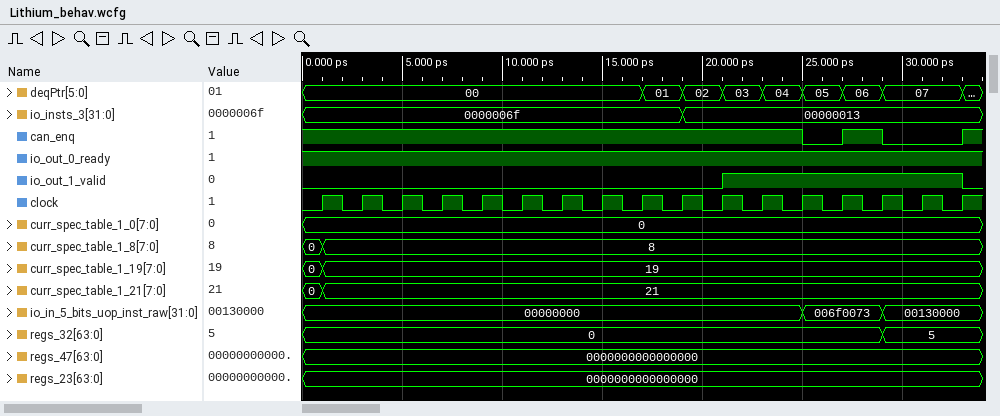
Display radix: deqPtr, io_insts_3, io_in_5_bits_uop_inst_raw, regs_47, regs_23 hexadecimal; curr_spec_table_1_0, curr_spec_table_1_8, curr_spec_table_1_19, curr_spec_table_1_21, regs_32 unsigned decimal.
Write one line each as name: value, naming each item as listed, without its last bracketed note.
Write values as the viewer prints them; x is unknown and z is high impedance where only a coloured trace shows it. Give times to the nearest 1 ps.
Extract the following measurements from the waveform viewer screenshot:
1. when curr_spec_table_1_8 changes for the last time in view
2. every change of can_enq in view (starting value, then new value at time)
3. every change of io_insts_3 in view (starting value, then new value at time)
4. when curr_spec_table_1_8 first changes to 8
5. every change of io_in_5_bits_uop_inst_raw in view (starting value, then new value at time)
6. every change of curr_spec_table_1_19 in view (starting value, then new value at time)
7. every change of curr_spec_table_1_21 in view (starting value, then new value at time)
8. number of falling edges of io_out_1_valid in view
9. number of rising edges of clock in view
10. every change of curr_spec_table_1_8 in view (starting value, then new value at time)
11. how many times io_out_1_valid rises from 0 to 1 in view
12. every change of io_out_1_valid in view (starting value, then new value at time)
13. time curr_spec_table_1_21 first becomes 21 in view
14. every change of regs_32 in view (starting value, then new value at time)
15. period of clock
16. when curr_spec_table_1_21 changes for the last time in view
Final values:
when curr_spec_table_1_8 changes for the last time in view: 1 ps
every change of can_enq in view: 1, 0 at 25 ps, 1 at 27 ps, 0 at 29 ps, 1 at 33 ps
every change of io_insts_3 in view: 0000006f, 00000013 at 19 ps
when curr_spec_table_1_8 first changes to 8: 1 ps
every change of io_in_5_bits_uop_inst_raw in view: 00000000, 006f0073 at 25 ps, 00130000 at 29 ps
every change of curr_spec_table_1_19 in view: 0, 19 at 1 ps
every change of curr_spec_table_1_21 in view: 0, 21 at 1 ps
number of falling edges of io_out_1_valid in view: 1
number of rising edges of clock in view: 17
every change of curr_spec_table_1_8 in view: 0, 8 at 1 ps
how many times io_out_1_valid rises from 0 to 1 in view: 1
every change of io_out_1_valid in view: 0, 1 at 21 ps, 0 at 33 ps
time curr_spec_table_1_21 first becomes 21 in view: 1 ps
every change of regs_32 in view: 0, 5 at 29 ps
period of clock: 2 ps
when curr_spec_table_1_21 changes for the last time in view: 1 ps
